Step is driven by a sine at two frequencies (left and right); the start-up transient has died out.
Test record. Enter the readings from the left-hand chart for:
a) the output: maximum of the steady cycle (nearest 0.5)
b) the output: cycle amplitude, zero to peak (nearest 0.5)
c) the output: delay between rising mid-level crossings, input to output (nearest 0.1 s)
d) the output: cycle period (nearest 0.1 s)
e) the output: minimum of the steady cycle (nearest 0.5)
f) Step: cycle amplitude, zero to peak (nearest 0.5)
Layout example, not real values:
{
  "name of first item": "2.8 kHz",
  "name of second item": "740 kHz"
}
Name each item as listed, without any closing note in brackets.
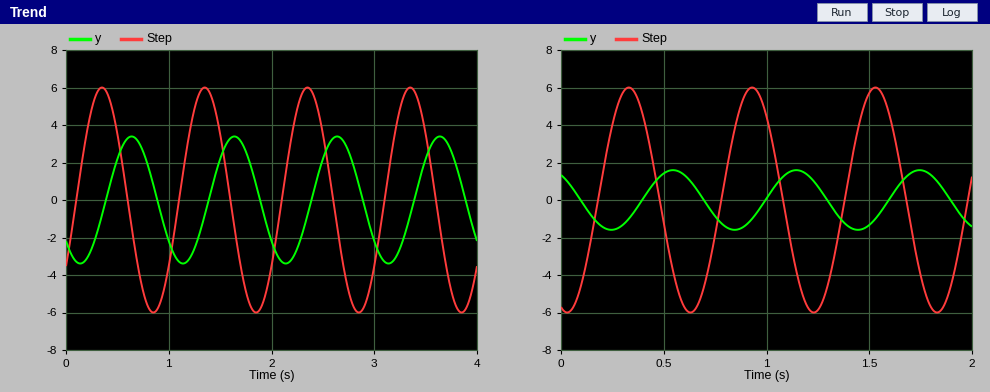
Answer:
{
  "the output: maximum of the steady cycle": "3.5",
  "the output: cycle amplitude, zero to peak": "3.5",
  "the output: delay between rising mid-level crossings, input to output": "0.3 s",
  "the output: cycle period": "1.0 s",
  "the output: minimum of the steady cycle": "-3.5",
  "Step: cycle amplitude, zero to peak": "6.0"
}
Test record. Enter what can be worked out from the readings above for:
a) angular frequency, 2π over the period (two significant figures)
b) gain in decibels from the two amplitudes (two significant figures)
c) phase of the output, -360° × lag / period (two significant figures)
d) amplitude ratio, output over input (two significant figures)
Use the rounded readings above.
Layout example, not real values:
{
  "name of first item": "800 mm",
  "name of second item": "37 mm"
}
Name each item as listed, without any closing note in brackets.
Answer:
{
  "angular frequency, 2π over the period": "6.3 rad/s",
  "gain in decibels from the two amplitudes": "-4.7 dB",
  "phase of the output, -360° × lag / period": "-110°",
  "amplitude ratio, output over input": "0.58"
}
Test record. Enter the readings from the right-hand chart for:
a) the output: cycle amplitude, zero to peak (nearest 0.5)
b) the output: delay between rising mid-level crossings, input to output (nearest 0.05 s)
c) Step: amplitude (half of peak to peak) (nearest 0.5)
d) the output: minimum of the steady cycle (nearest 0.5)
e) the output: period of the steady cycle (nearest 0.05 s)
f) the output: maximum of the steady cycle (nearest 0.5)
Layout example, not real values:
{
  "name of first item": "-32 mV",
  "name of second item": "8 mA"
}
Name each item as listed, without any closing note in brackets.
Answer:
{
  "the output: cycle amplitude, zero to peak": "1.5",
  "the output: delay between rising mid-level crossings, input to output": "0.20 s",
  "Step: amplitude (half of peak to peak)": "6.0",
  "the output: minimum of the steady cycle": "-1.5",
  "the output: period of the steady cycle": "0.60 s",
  "the output: maximum of the steady cycle": "1.5"
}
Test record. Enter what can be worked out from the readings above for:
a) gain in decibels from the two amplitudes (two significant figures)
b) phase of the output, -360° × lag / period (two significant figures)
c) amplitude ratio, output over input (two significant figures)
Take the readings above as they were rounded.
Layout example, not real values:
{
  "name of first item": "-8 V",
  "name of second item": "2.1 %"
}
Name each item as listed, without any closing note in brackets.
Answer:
{
  "gain in decibels from the two amplitudes": "-12 dB",
  "phase of the output, -360° × lag / period": "-120°",
  "amplitude ratio, output over input": "0.25"
}
